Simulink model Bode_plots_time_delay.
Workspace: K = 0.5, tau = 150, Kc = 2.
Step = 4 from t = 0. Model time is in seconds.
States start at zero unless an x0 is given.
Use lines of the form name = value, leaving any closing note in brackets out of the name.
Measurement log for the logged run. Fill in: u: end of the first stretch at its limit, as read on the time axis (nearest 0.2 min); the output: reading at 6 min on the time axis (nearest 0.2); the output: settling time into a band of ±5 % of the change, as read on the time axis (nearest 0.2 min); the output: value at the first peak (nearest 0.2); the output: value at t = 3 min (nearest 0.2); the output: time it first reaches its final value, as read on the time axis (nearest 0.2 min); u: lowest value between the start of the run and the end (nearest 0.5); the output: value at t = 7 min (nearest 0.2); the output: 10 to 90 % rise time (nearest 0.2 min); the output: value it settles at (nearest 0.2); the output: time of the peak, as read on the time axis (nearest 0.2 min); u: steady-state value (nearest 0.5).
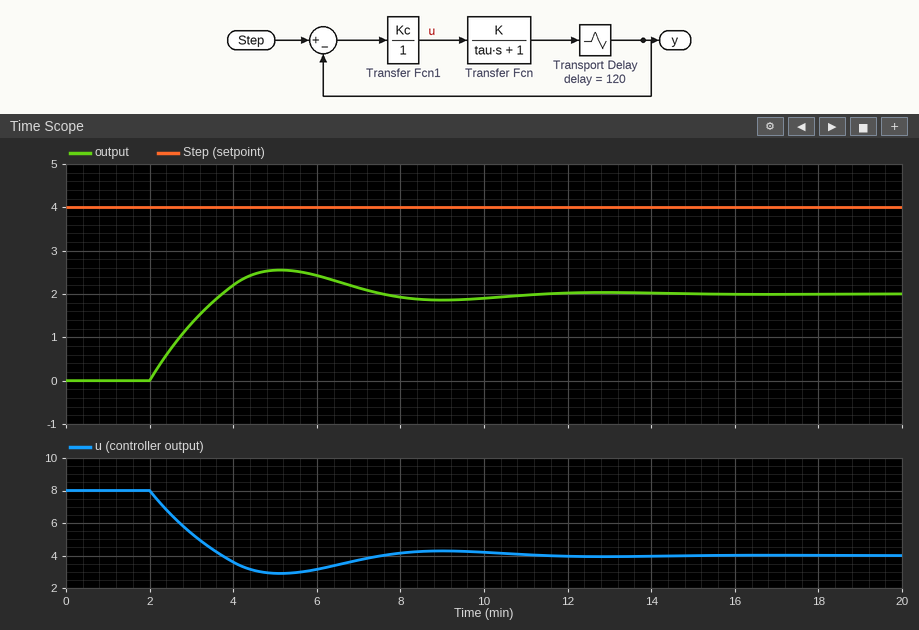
u: end of the first stretch at its limit, as read on the time axis = 2.0 min
the output: reading at 6 min on the time axis = 2.4
the output: settling time into a band of ±5 % of the change, as read on the time axis = 10.0 min
the output: value at the first peak = 2.6
the output: value at t = 3 min = 1.4
the output: time it first reaches its final value, as read on the time axis = 3.8 min
u: lowest value between the start of the run and the end = 3.0
the output: value at t = 7 min = 2.2
the output: 10 to 90 % rise time = 1.4 min
the output: value it settles at = 2.0
the output: time of the peak, as read on the time axis = 5.2 min
u: steady-state value = 4.0
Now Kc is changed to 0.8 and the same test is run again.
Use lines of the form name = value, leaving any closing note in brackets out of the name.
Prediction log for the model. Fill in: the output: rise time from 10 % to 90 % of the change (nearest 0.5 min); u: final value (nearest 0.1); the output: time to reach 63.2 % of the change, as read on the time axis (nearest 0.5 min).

the output: rise time from 10 % to 90 % of the change = 2.5 min
u: final value = 2.3
the output: time to reach 63.2 % of the change, as read on the time axis = 3.5 min
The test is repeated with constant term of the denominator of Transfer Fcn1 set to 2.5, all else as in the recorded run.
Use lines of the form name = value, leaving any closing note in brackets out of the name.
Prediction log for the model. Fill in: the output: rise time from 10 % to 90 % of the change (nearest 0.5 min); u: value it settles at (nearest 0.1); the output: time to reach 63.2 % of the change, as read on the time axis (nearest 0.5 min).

the output: rise time from 10 % to 90 % of the change = 2.5 min
u: value it settles at = 2.3
the output: time to reach 63.2 % of the change, as read on the time axis = 3.5 min
